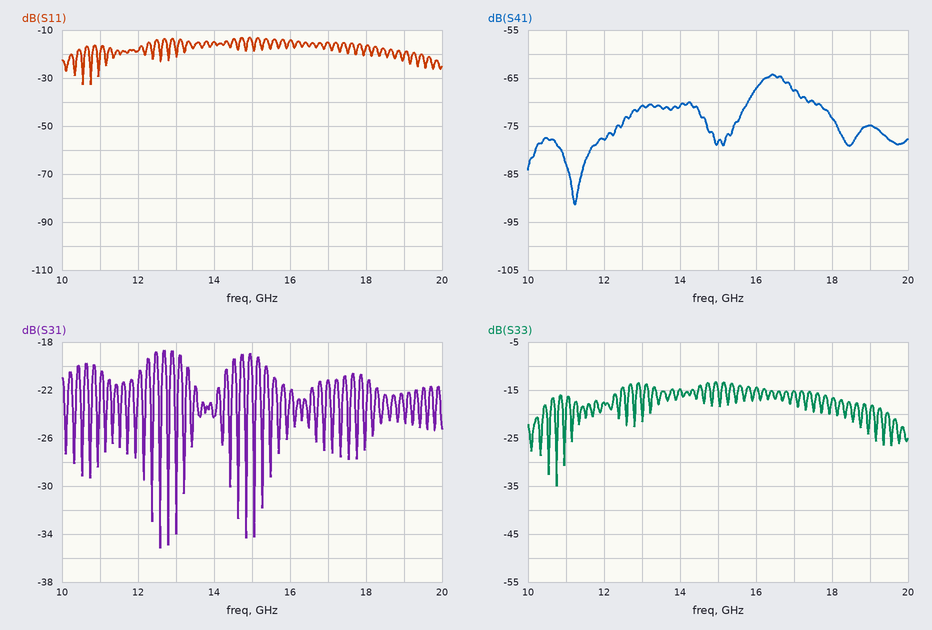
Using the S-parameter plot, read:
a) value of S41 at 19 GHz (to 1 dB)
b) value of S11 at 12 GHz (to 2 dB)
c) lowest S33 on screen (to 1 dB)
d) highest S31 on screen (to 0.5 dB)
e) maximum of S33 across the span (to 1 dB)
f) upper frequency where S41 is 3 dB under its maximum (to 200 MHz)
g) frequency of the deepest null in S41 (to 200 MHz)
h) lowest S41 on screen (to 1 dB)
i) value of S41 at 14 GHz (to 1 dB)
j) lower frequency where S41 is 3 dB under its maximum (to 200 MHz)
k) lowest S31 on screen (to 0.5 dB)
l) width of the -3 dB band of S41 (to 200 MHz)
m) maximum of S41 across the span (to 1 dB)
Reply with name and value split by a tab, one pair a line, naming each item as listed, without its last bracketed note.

value of S41 at 19 GHz	-75 dB
value of S11 at 12 GHz	-18 dB
lowest S33 on screen	-35 dB
highest S31 on screen	-18.5 dB
maximum of S33 across the span	-13 dB
upper frequency where S41 is 3 dB under its maximum	17.0 GHz
frequency of the deepest null in S41	11.2 GHz
lowest S41 on screen	-91 dB
value of S41 at 14 GHz	-71 dB
lower frequency where S41 is 3 dB under its maximum	16.0 GHz
lowest S31 on screen	-35.0 dB
width of the -3 dB band of S41	1.0 GHz
maximum of S41 across the span	-64 dB
